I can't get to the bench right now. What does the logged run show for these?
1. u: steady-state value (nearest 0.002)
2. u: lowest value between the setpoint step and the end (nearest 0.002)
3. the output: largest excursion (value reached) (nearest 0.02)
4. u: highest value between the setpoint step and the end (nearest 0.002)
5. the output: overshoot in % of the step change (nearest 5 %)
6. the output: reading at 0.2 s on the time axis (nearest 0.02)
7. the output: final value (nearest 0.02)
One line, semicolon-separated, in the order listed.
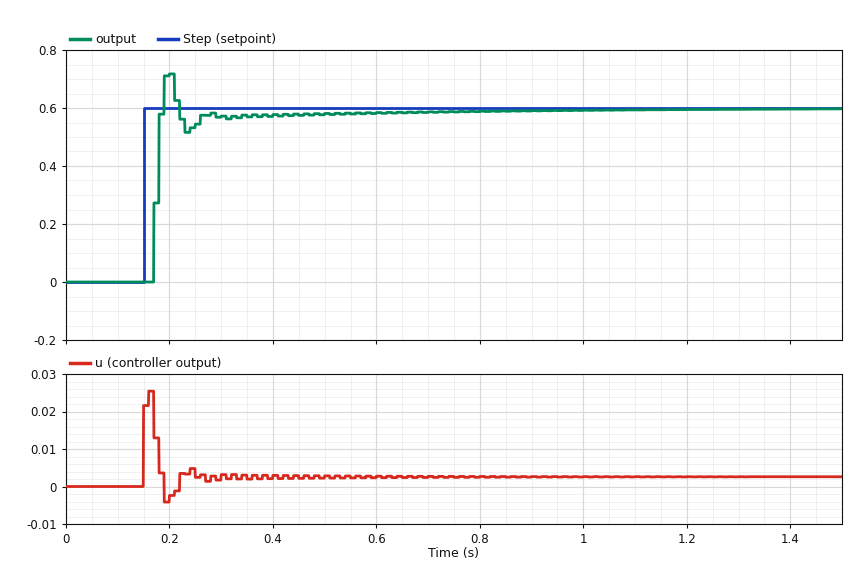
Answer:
0.002; -0.004; 0.72; 0.026; 20 %; 0.72; 0.60
